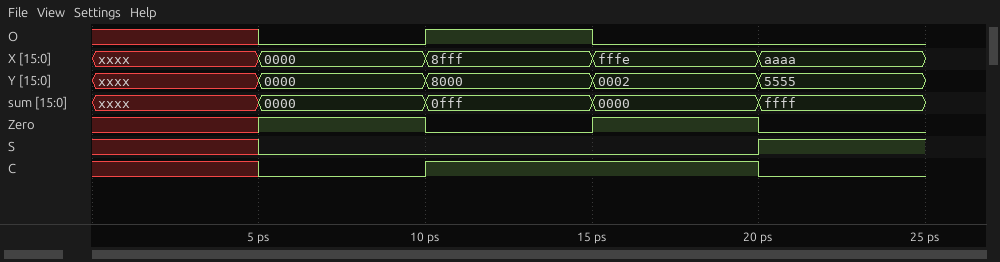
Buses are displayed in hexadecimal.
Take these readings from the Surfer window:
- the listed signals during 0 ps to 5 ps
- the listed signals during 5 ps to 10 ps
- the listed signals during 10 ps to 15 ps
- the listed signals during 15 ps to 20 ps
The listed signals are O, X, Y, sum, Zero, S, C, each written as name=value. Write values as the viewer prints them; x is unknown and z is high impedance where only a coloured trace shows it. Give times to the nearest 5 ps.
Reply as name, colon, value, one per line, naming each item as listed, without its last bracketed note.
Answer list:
the listed signals during 0 ps to 5 ps: O=x, X=xxxx, Y=xxxx, sum=xxxx, Zero=x, S=x, C=x
the listed signals during 5 ps to 10 ps: O=0, X=0000, Y=0000, sum=0000, Zero=1, S=0, C=0
the listed signals during 10 ps to 15 ps: O=1, X=8fff, Y=8000, sum=0fff, Zero=0, S=0, C=1
the listed signals during 15 ps to 20 ps: O=0, X=fffe, Y=0002, sum=0000, Zero=1, S=0, C=1
